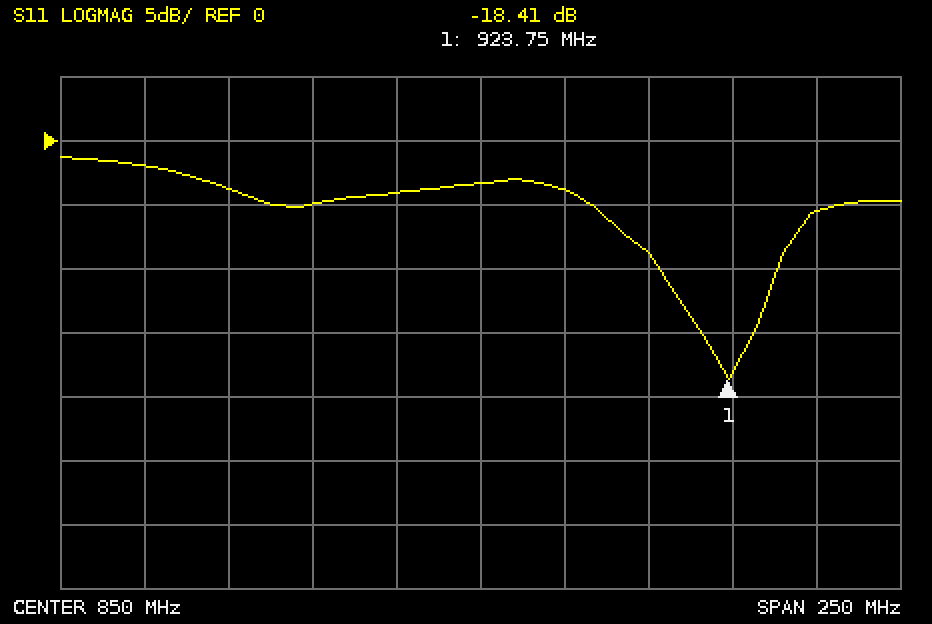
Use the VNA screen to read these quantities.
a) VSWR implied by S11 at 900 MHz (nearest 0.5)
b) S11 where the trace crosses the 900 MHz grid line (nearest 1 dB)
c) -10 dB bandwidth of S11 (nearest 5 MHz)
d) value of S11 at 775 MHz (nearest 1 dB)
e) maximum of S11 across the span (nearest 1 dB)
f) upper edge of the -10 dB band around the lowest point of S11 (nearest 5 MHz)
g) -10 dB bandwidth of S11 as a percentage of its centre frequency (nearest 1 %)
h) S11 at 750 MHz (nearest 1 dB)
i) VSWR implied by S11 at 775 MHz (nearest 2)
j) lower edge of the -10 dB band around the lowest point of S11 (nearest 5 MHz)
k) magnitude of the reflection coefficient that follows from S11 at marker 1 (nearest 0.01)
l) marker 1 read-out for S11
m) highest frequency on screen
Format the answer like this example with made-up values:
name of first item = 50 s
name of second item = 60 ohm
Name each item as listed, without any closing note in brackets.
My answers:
VSWR implied by S11 at 900 MHz = 2.0
S11 where the trace crosses the 900 MHz grid line = -9 dB
-10 dB bandwidth of S11 = 35 MHz
value of S11 at 775 MHz = -4 dB
maximum of S11 across the span = -1 dB
upper edge of the -10 dB band around the lowest point of S11 = 940 MHz
-10 dB bandwidth of S11 as a percentage of its centre frequency = 4 %
S11 at 750 MHz = -2 dB
VSWR implied by S11 at 775 MHz = 4
lower edge of the -10 dB band around the lowest point of S11 = 905 MHz
magnitude of the reflection coefficient that follows from S11 at marker 1 = 0.12
marker 1 read-out for S11 = -18.41 dB
highest frequency on screen = 975 MHz
